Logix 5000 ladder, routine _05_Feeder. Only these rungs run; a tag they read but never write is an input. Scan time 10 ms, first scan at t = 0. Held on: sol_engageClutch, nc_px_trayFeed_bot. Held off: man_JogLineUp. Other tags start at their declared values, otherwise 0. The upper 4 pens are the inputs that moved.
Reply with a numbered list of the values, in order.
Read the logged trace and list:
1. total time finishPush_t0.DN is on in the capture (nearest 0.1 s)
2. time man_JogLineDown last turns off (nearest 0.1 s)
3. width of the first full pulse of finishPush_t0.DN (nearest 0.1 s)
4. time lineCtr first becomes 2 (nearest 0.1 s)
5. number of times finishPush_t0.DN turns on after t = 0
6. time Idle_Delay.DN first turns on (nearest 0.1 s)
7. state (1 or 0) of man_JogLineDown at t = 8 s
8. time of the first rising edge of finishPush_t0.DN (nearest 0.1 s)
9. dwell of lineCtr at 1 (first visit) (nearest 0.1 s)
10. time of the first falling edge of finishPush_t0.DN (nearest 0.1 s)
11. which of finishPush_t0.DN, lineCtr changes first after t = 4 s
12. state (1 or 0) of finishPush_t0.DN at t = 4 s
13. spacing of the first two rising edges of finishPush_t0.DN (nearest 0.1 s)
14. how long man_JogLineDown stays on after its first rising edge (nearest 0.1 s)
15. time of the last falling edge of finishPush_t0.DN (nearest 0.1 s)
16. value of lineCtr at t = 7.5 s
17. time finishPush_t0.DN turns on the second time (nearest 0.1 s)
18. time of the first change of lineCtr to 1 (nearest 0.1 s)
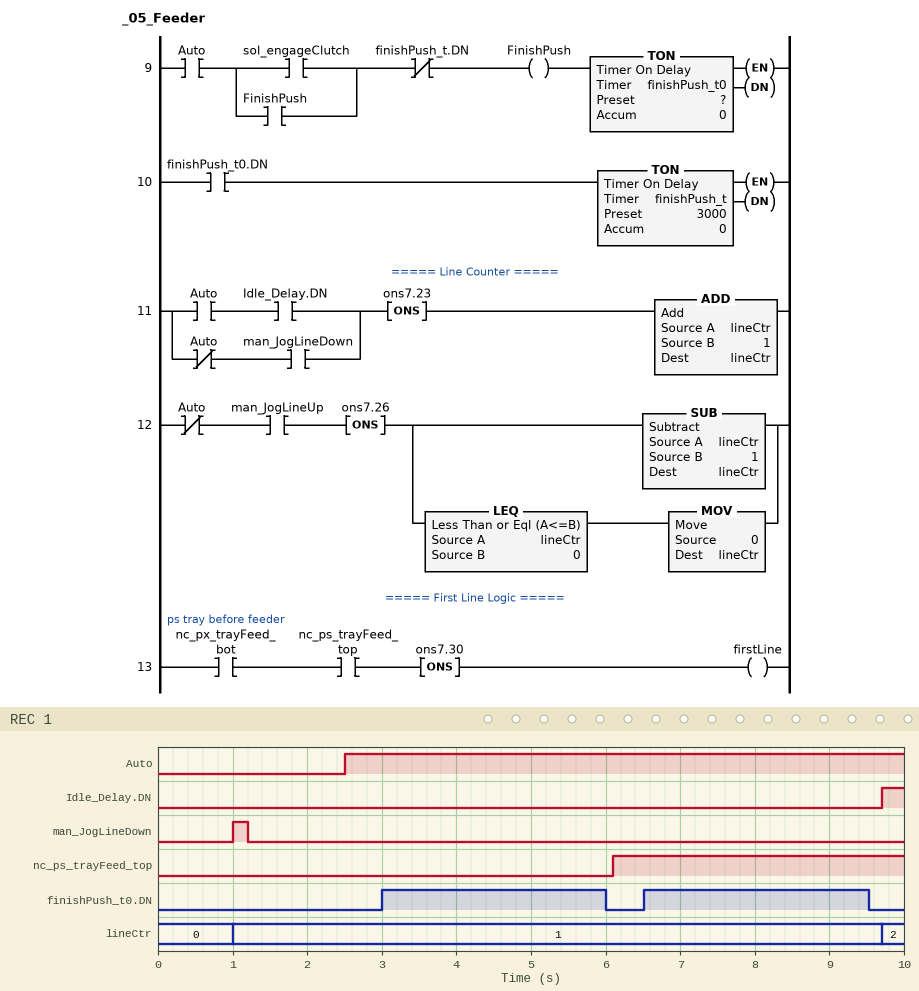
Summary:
1. 6.0 s
2. 1.2 s
3. 3.0 s
4. 9.7 s
5. 2
6. 9.7 s
7. 0
8. 3.0 s
9. 8.7 s
10. 6.0 s
11. finishPush_t0.DN
12. 1
13. 3.5 s
14. 0.2 s
15. 9.5 s
16. 1
17. 6.5 s
18. 1.0 s
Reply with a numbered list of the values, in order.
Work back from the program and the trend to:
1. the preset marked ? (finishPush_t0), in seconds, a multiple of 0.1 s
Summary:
1. 0.5 s
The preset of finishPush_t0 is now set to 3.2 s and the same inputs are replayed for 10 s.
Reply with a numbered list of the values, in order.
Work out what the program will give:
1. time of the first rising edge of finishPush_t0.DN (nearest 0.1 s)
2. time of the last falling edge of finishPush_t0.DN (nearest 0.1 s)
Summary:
1. 5.7 s
2. 8.7 s
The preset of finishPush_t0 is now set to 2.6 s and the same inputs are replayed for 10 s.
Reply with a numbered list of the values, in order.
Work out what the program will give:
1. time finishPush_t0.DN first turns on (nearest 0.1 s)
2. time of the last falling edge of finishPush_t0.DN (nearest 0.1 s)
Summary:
1. 5.1 s
2. 8.1 s
